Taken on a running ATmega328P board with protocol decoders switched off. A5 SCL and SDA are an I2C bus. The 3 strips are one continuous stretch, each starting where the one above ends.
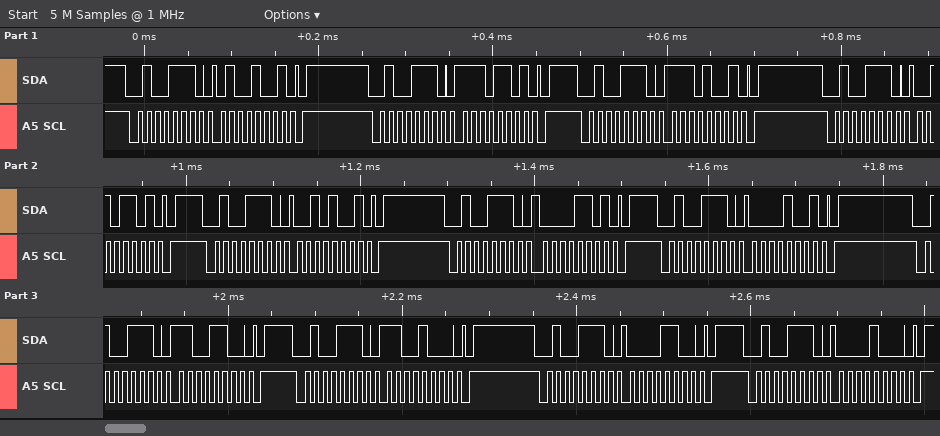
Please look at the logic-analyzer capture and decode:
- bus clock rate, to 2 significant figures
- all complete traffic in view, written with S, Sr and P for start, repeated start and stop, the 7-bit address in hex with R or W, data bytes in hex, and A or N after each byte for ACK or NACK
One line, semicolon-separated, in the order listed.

100 kHz; S 27W A 49 A P S 27W A ED A P S 27W A E9 A P S 27W A 2D A P S 27W A 29 A P S 27W A 0D A P S 27W A 09 A P S 27W A CC A P S 27W A C8 A P S 27W A 0C A P S 27W A 08 A P
